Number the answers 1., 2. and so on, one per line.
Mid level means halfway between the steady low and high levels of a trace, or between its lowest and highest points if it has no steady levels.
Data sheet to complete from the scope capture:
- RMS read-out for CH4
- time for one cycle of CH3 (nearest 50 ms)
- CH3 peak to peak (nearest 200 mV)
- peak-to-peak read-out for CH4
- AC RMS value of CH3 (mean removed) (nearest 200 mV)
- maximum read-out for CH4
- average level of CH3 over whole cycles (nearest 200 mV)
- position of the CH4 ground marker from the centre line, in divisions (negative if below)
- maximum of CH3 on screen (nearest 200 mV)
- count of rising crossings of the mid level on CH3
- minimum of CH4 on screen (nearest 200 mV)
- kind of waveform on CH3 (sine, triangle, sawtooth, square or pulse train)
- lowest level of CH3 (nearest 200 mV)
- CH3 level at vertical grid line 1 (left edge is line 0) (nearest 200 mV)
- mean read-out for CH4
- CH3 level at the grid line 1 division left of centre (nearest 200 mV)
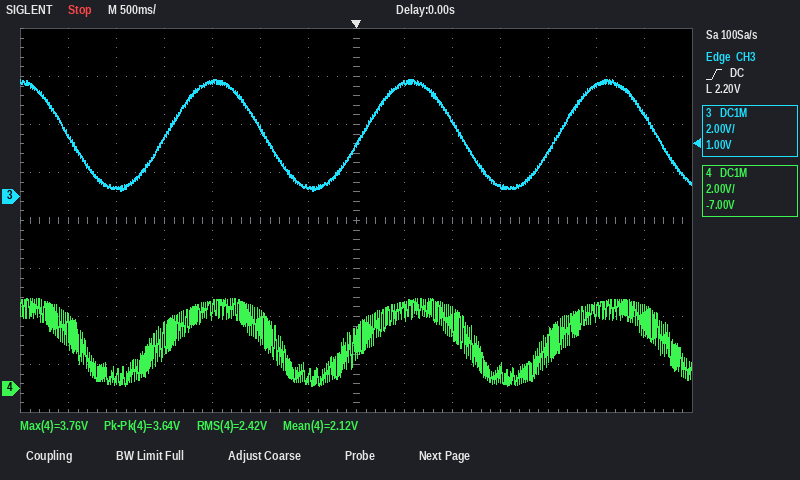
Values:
1. 2.42 V
2. 2.05 s
3. 4.6 V
4. 3.64 V
5. 1.6 V
6. 3.76 V
7. 2.6 V
8. -3.5 div
9. 4.8 V
10. 3
11. 200 mV
12. sine
13. 200 mV
14. 2.6 V
15. 2.12 V
16. 400 mV
